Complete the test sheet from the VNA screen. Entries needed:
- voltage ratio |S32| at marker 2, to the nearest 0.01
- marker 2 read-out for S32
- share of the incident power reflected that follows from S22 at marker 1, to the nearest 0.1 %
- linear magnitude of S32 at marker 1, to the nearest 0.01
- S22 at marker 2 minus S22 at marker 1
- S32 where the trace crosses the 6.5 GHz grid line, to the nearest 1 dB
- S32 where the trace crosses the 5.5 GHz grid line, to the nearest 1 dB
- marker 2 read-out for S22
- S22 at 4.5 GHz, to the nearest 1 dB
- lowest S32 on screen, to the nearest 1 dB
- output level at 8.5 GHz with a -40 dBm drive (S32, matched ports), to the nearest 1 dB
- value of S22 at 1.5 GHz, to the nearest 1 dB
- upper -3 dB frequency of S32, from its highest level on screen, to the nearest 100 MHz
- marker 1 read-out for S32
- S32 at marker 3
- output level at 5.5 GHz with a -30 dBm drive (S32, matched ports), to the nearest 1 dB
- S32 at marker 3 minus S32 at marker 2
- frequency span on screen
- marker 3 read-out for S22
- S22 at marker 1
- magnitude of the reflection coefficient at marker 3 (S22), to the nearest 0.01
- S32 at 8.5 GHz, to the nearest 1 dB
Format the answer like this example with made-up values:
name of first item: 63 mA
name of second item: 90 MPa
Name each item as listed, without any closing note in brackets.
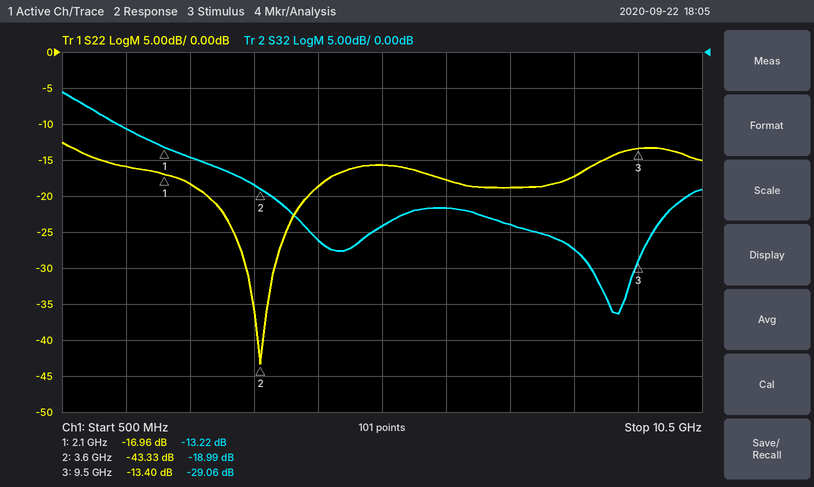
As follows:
voltage ratio |S32| at marker 2, to the nearest 0.01: 0.11
marker 2 read-out for S32: -18.99 dB
share of the incident power reflected that follows from S22 at marker 1, to the nearest 0.1 %: 2.0 %
linear magnitude of S32 at marker 1, to the nearest 0.01: 0.22
S22 at marker 2 minus S22 at marker 1: -26.37 dB
S32 where the trace crosses the 6.5 GHz grid line, to the nearest 1 dB: -22 dB
S32 where the trace crosses the 5.5 GHz grid line, to the nearest 1 dB: -24 dB
marker 2 read-out for S22: -43.33 dB
S22 at 4.5 GHz, to the nearest 1 dB: -19 dB
lowest S32 on screen, to the nearest 1 dB: -36 dB
output level at 8.5 GHz with a -40 dBm drive (S32, matched ports), to the nearest 1 dB: -67 dBm
value of S22 at 1.5 GHz, to the nearest 1 dB: -16 dB
upper -3 dB frequency of S32, from its highest level on screen, to the nearest 100 MHz: 1.1 GHz
marker 1 read-out for S32: -13.22 dB
S32 at marker 3: -29.06 dB
output level at 5.5 GHz with a -30 dBm drive (S32, matched ports), to the nearest 1 dB: -54 dBm
S32 at marker 3 minus S32 at marker 2: -10.07 dB
frequency span on screen: 10 GHz
marker 3 read-out for S22: -13.40 dB
S22 at marker 1: -16.96 dB
magnitude of the reflection coefficient at marker 3 (S22), to the nearest 0.01: 0.21
S32 at 8.5 GHz, to the nearest 1 dB: -27 dB
